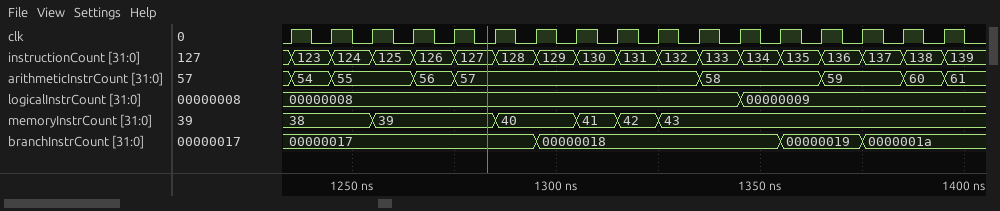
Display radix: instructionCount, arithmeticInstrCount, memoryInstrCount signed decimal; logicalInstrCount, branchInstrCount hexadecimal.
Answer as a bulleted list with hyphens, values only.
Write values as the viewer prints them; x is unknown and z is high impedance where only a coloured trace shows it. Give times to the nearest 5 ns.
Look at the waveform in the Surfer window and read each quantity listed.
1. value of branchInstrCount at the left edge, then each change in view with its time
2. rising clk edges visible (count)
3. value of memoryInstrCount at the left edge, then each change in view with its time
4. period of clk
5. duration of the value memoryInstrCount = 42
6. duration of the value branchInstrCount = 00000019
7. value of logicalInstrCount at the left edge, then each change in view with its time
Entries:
- 00000017, 00000018 at 1295 ns, 00000019 at 1355 ns, 0000001a at 1375 ns
- 17
- 38, 39 at 1255 ns, 40 at 1285 ns, 41 at 1305 ns, 42 at 1315 ns, 43 at 1325 ns
- 10 ns
- 10 ns
- 20 ns
- 00000008, 00000009 at 1345 ns
